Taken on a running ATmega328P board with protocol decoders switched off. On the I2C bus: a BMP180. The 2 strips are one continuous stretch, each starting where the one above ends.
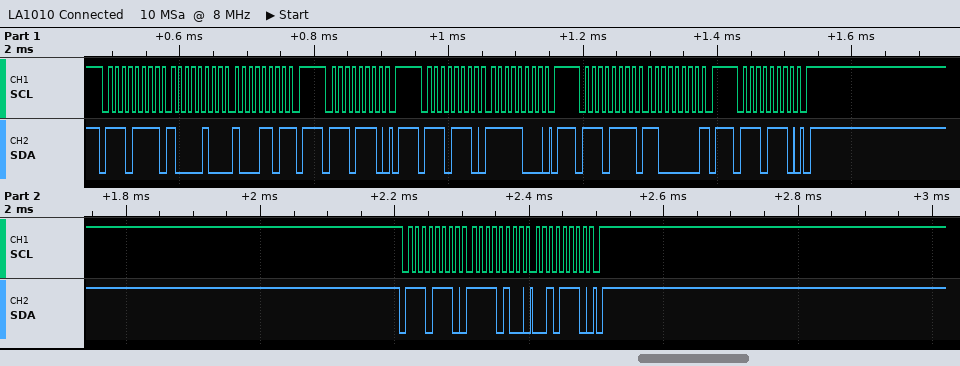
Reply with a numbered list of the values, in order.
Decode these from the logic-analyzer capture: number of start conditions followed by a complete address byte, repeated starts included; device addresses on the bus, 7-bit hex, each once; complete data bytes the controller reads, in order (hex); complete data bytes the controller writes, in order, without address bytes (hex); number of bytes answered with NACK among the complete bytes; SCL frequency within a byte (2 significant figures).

1. 6
2. 0x77
3. 84 8D C0
4. F8 F4 2E
5. 2
6. 100 kHz
